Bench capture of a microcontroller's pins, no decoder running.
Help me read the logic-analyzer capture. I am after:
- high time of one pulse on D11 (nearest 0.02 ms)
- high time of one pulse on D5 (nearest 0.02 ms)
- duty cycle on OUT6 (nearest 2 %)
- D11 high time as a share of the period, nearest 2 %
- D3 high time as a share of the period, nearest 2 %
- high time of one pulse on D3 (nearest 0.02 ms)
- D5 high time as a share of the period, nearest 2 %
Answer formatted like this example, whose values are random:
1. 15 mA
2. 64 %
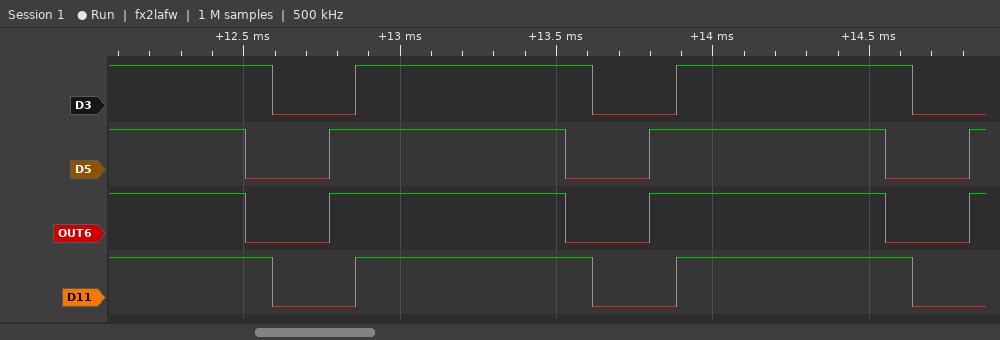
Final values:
1. 0.76 ms
2. 0.76 ms
3. 74 %
4. 74 %
5. 74 %
6. 0.76 ms
7. 74 %
